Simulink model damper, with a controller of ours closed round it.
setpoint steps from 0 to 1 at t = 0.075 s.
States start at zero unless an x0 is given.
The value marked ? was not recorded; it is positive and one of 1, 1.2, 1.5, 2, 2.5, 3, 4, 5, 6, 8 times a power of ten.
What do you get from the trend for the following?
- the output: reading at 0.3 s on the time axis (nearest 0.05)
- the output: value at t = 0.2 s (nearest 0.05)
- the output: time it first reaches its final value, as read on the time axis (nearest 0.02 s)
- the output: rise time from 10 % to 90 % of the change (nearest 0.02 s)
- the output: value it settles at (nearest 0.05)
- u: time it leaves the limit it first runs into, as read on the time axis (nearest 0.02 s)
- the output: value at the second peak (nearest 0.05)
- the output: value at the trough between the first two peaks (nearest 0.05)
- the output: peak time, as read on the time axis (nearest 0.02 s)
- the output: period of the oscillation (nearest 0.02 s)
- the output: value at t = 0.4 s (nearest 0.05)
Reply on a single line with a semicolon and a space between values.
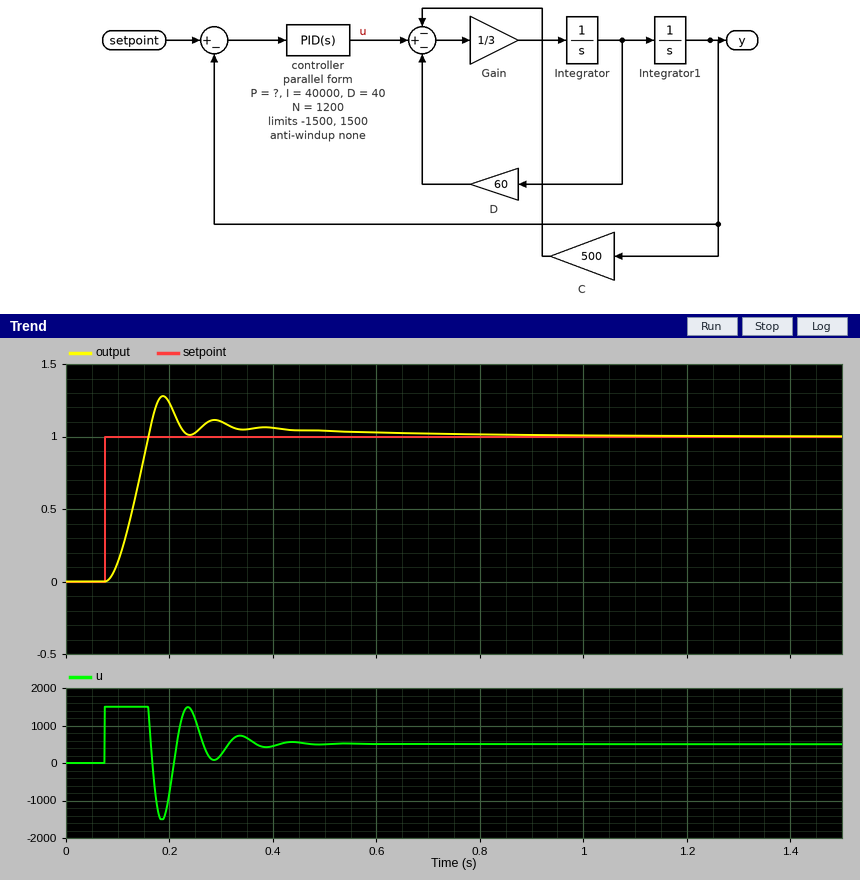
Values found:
1.10; 1.25; 0.16 s; 0.06 s; 1.00; 0.16 s; 1.10; 1.00; 0.18 s; 0.10 s; 1.05
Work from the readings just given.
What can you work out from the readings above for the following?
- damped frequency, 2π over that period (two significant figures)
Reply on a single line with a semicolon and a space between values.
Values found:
63 rad/s
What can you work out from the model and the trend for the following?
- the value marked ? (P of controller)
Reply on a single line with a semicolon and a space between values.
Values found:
12000
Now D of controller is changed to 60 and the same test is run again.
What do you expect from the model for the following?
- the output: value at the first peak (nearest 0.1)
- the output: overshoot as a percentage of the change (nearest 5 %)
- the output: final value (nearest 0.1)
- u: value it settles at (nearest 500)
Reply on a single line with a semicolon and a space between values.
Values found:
1.3; 25 %; 1.0; 500
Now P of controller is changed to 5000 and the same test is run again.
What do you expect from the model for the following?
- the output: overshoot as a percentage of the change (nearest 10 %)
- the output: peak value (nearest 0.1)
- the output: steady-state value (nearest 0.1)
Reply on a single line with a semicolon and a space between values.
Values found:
40 %; 1.4; 1.0
